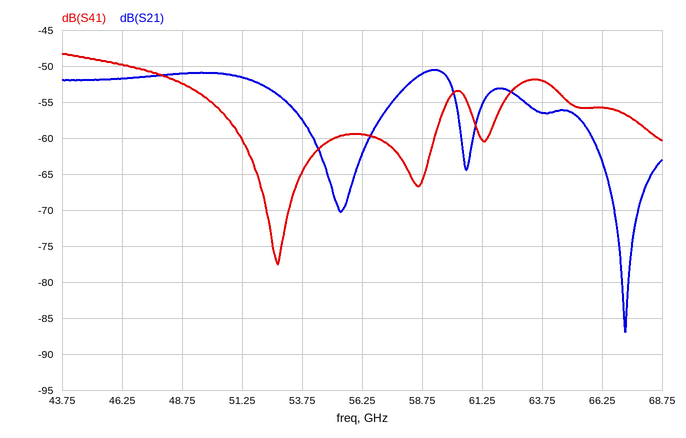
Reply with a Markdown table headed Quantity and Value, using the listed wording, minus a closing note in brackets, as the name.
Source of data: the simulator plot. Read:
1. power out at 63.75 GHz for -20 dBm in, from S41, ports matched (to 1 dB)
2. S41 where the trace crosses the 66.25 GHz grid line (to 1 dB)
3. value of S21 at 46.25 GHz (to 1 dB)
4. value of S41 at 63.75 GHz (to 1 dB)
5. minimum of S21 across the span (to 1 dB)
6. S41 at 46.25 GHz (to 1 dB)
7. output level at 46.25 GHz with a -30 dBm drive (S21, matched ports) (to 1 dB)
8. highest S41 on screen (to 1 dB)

| Quantity | Value |
|---|---|
| power out at 63.75 GHz for -20 dBm in, from S41, ports matched | -72 dBm |
| S41 where the trace crosses the 66.25 GHz grid line | -56 dB |
| value of S21 at 46.25 GHz | -52 dB |
| value of S41 at 63.75 GHz | -52 dB |
| minimum of S21 across the span | -87 dB |
| S41 at 46.25 GHz | -50 dB |
| output level at 46.25 GHz with a -30 dBm drive (S21, matched ports) | -82 dBm |
| highest S41 on screen | -48 dB |
